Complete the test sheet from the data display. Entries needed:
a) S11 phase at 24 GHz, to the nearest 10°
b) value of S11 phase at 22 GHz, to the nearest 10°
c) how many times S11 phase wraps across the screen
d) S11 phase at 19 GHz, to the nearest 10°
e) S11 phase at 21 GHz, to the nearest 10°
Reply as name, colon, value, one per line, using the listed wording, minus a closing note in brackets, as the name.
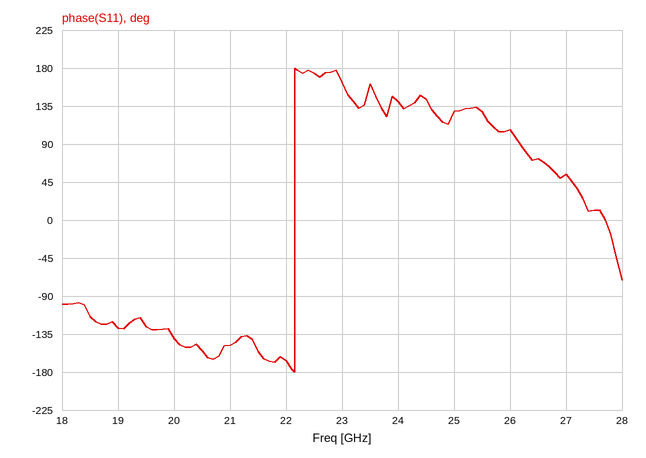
S11 phase at 24 GHz, to the nearest 10°: 140°
value of S11 phase at 22 GHz, to the nearest 10°: -170°
how many times S11 phase wraps across the screen: 1
S11 phase at 19 GHz, to the nearest 10°: -130°
S11 phase at 21 GHz, to the nearest 10°: -150°
